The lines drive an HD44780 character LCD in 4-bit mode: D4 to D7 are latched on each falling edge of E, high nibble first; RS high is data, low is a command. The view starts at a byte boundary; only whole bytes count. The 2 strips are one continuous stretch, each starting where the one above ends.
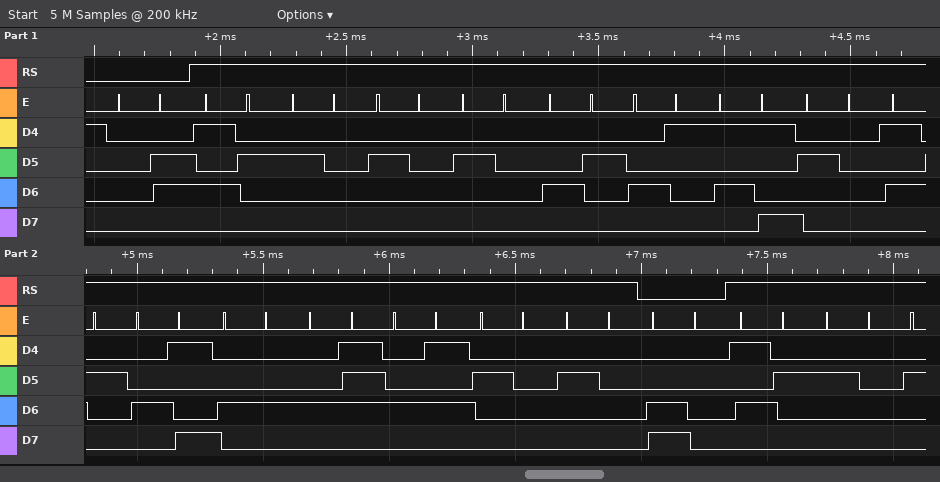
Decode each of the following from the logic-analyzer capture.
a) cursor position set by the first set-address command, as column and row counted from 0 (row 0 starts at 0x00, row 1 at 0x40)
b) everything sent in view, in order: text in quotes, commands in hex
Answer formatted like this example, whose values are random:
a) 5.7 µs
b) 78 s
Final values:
a) column 0, row 1
b) 0x06 "R   BAY RIDGE  " 0xC0 "R "
